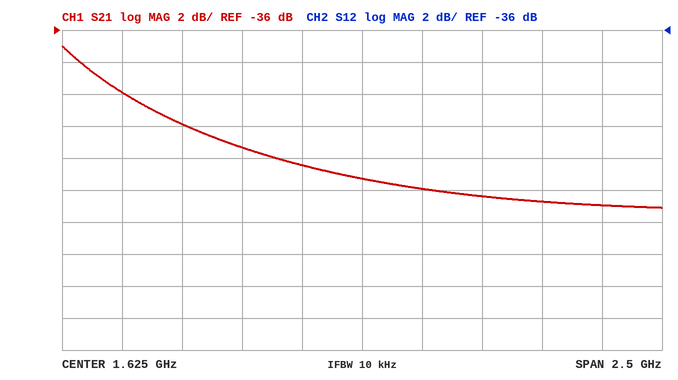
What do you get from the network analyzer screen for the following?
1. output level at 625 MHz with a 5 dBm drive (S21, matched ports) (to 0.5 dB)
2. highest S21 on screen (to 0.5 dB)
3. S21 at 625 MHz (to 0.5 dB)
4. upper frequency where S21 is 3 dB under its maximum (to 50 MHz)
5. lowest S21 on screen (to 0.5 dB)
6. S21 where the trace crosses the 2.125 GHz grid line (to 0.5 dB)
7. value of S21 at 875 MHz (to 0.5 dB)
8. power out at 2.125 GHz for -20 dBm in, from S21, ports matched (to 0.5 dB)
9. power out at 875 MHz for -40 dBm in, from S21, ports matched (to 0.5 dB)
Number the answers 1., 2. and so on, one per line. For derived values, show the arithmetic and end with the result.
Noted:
1. 5 dBm + (-40.0 dB) = -35.0 dBm
2. -37.0 dB
3. -40.0 dB
4. 650 MHz
5. -47.0 dB
6. -46.5 dB
7. -42.0 dB
8. -20 dBm + (-46.5 dB) = -66.5 dBm
9. -40 dBm + (-42.0 dB) = -82.0 dBm
